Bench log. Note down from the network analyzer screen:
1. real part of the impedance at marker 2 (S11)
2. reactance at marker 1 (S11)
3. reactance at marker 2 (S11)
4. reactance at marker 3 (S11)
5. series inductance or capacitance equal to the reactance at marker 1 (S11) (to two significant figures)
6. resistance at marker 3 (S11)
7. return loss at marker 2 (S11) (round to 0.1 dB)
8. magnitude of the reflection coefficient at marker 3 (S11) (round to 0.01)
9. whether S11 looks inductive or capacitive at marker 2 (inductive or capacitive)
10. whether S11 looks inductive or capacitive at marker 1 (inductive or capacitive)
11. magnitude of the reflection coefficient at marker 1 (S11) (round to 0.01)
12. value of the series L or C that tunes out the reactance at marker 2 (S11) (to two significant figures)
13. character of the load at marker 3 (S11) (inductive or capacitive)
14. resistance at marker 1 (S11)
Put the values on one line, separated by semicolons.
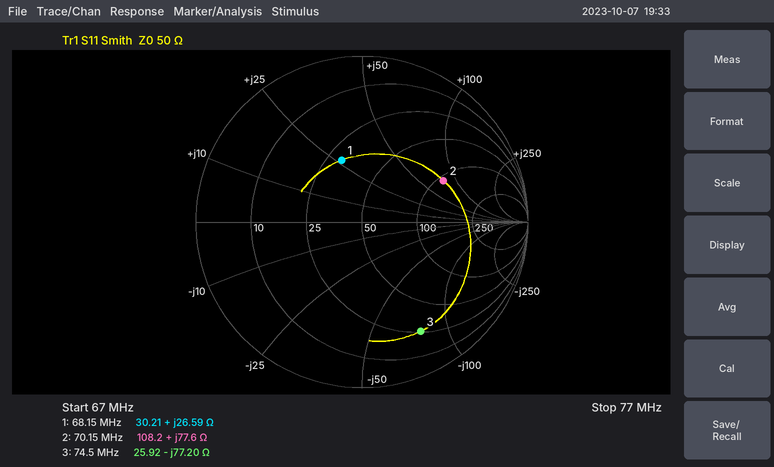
108.2 Ω; +26.59 Ω; +77.6 Ω; -77.20 Ω; 62 nH; 25.92 Ω; 5.2 dB; 0.75; inductive; inductive; 0.39; 29 pF; capacitive; 30.21 Ω
